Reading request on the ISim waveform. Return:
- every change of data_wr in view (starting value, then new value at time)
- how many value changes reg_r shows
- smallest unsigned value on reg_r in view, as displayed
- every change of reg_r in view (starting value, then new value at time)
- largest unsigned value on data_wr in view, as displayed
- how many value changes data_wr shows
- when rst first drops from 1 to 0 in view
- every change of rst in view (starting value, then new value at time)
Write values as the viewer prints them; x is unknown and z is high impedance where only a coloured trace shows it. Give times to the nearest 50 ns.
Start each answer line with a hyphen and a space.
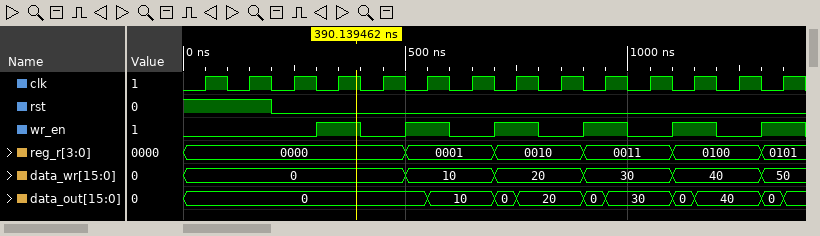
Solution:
- 0, 10 at 500 ns, 20 at 700 ns, 30 at 900 ns, 40 at 1100 ns, 50 at 1300 ns
- 5
- 0000
- 0000, 0001 at 500 ns, 0010 at 700 ns, 0011 at 900 ns, 0100 at 1100 ns, 0101 at 1300 ns
- 50
- 5
- 200 ns
- 1, 0 at 200 ns
